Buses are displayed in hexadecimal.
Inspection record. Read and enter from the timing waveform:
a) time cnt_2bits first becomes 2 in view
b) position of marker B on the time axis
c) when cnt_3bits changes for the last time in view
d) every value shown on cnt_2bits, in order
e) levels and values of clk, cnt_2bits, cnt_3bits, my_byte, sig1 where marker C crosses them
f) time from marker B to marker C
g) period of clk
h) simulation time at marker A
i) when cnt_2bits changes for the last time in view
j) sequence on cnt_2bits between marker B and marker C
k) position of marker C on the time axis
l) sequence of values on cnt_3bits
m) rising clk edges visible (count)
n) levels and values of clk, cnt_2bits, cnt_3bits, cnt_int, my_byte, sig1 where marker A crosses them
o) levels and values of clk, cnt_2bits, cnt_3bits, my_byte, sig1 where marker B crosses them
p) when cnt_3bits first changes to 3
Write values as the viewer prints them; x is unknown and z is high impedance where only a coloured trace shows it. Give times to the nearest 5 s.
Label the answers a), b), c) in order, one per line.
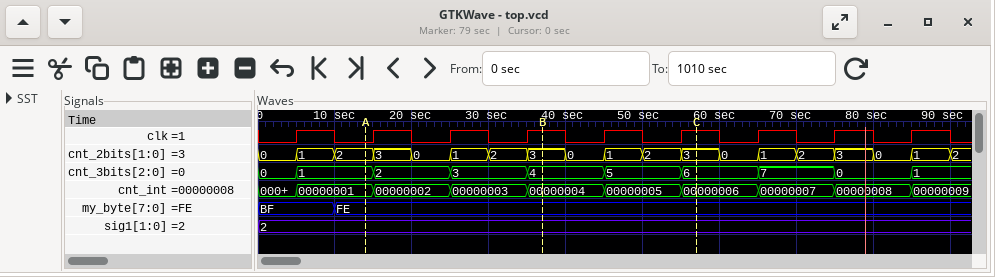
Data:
a) 10 s
b) 35 s
c) 85 s
d) 0, 1, 2, 3, 0, 1, 2, 3, 0, 1, 2, 3, 0, 1, 2, 3, 0, 1, 2
e) clk=1, cnt_2bits=3, cnt_3bits=6, my_byte=FE, sig1=2
f) 20 s
g) 10 s
h) 15 s
i) 90 s
j) 3, 0, 1, 2, 3
k) 55 s
l) 0, 1, 2, 3, 4, 5, 6, 7, 0, 1
m) 9
n) clk=0, cnt_2bits=2, cnt_3bits=1, cnt_int=00000001, my_byte=FE, sig1=2
o) clk=1, cnt_2bits=3, cnt_3bits=4, my_byte=FE, sig1=2
p) 25 s
